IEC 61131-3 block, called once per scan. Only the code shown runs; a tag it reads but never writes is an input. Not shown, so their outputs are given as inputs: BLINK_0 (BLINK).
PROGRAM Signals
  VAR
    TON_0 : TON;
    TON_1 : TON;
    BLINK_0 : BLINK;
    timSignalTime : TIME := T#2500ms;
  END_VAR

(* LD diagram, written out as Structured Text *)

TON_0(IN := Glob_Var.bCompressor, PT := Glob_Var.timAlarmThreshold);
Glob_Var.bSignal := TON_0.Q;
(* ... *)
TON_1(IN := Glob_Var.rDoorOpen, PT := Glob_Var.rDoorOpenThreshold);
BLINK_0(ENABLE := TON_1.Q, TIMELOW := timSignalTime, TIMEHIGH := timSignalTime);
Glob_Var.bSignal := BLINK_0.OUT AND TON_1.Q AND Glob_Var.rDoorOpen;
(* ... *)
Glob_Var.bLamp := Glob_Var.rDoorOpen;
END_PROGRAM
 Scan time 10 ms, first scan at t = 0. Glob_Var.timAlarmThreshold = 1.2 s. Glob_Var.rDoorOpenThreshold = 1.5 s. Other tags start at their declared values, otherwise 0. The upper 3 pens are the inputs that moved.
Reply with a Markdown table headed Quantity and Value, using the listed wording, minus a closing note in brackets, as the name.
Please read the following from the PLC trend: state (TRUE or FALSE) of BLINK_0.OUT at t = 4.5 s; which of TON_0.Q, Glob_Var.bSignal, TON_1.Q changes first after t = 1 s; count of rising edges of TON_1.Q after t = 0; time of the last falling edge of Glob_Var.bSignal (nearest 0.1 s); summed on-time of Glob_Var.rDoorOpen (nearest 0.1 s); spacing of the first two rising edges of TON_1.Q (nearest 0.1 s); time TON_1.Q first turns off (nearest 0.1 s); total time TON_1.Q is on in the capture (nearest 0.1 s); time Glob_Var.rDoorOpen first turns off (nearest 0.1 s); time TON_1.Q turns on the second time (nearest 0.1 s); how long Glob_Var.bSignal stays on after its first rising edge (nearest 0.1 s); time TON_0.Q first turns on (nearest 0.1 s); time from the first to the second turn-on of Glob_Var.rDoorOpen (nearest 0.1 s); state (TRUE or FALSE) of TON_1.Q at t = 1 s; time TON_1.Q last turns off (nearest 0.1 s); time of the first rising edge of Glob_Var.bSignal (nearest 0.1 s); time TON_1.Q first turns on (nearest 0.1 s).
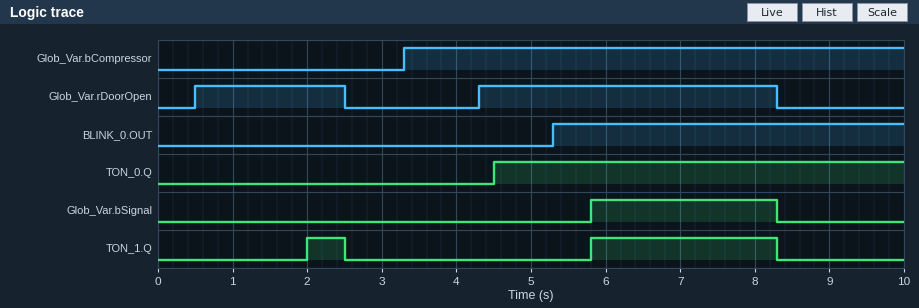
| Quantity | Value |
|---|---|
| state (TRUE or FALSE) of BLINK_0.OUT at t = 4.5 s | FALSE |
| which of TON_0.Q, Glob_Var.bSignal, TON_1.Q changes first after t = 1 s | TON_1.Q |
| count of rising edges of TON_1.Q after t = 0 | 2 |
| time of the last falling edge of Glob_Var.bSignal | 8.3 s |
| summed on-time of Glob_Var.rDoorOpen | 6.0 s |
| spacing of the first two rising edges of TON_1.Q | 3.8 s |
| time TON_1.Q first turns off | 2.5 s |
| total time TON_1.Q is on in the capture | 3.0 s |
| time Glob_Var.rDoorOpen first turns off | 2.5 s |
| time TON_1.Q turns on the second time | 5.8 s |
| how long Glob_Var.bSignal stays on after its first rising edge | 2.5 s |
| time TON_0.Q first turns on | 4.5 s |
| time from the first to the second turn-on of Glob_Var.rDoorOpen | 3.8 s |
| state (TRUE or FALSE) of TON_1.Q at t = 1 s | FALSE |
| time TON_1.Q last turns off | 8.3 s |
| time of the first rising edge of Glob_Var.bSignal | 5.8 s |
| time TON_1.Q first turns on | 2.0 s |
